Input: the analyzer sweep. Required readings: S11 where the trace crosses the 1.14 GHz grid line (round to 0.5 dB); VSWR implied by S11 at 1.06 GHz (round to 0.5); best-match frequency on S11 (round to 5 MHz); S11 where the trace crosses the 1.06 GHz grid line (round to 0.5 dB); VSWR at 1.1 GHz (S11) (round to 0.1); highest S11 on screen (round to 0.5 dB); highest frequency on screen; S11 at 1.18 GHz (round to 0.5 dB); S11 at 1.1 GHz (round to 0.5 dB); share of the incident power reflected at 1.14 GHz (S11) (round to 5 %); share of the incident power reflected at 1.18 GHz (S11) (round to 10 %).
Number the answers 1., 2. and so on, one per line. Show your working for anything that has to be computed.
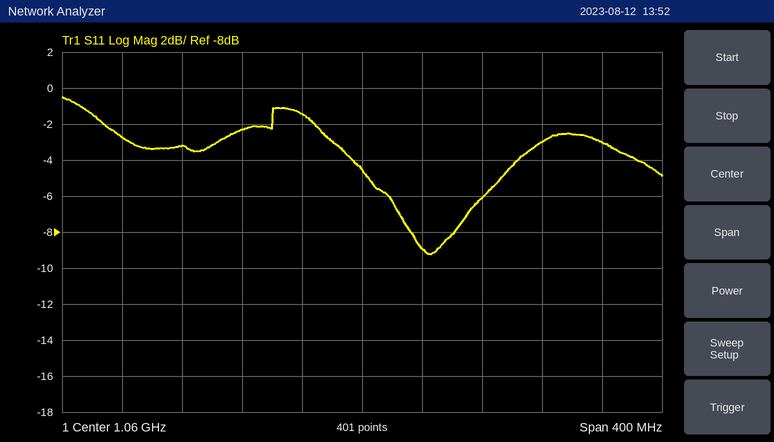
1. -6.0 dB
2. |Γ| = 10^(-4.5/20) = 0.5957; VSWR = (1 + 0.5957)/(1 − 0.5957) ≈ 4.0
3. 1.105 GHz
4. -4.5 dB
5. |Γ| = 10^(-9/20) = 0.3548; VSWR = (1 + 0.3548)/(1 − 0.3548) ≈ 2.1
6. -0.5 dB
7. 1.26 GHz
8. -3.0 dB
9. -9.0 dB
10. 10^(-6/10) ≈ 25 %
11. 10^(-3/10) ≈ 50 %
